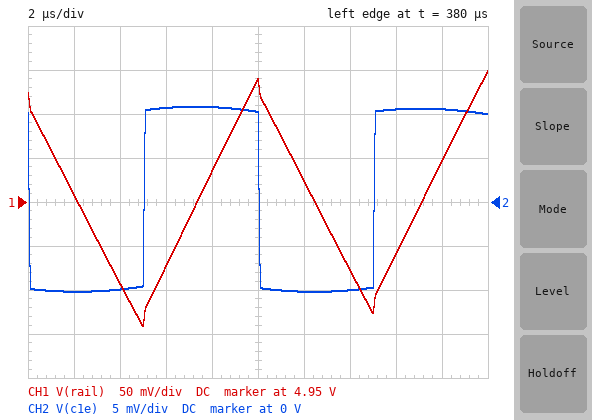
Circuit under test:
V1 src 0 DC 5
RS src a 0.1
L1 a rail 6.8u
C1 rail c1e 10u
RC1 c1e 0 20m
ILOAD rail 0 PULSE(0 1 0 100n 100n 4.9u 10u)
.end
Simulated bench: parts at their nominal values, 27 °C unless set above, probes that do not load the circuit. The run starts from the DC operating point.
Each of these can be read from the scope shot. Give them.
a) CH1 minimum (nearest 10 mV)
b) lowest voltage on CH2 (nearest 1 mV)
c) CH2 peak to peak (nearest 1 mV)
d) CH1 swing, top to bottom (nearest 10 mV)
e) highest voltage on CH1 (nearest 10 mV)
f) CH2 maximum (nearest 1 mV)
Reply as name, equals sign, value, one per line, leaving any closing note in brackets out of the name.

CH1 minimum = 4.81 V
lowest voltage on CH2 = -10 mV
CH2 peak to peak = 21 mV
CH1 swing, top to bottom = 290 mV
highest voltage on CH1 = 5.10 V
CH2 maximum = 11 mV
